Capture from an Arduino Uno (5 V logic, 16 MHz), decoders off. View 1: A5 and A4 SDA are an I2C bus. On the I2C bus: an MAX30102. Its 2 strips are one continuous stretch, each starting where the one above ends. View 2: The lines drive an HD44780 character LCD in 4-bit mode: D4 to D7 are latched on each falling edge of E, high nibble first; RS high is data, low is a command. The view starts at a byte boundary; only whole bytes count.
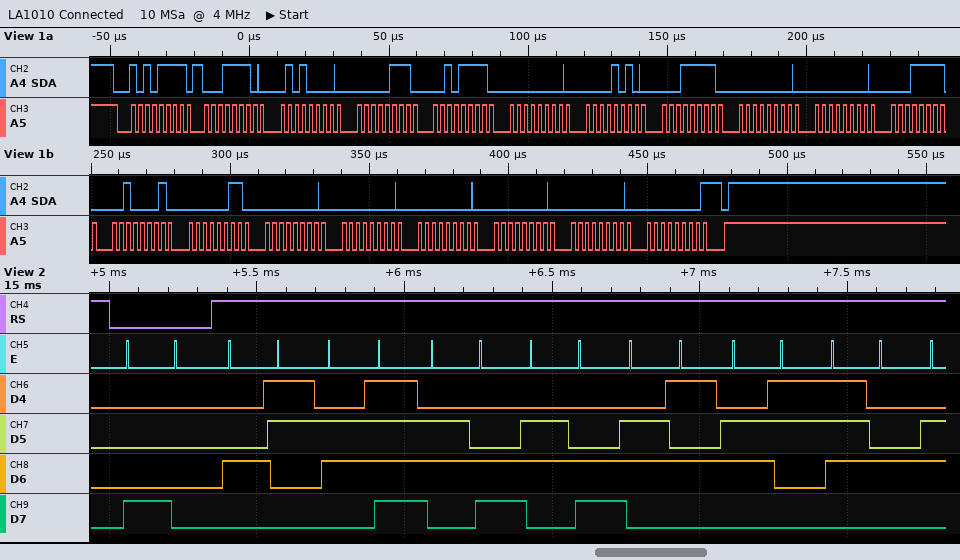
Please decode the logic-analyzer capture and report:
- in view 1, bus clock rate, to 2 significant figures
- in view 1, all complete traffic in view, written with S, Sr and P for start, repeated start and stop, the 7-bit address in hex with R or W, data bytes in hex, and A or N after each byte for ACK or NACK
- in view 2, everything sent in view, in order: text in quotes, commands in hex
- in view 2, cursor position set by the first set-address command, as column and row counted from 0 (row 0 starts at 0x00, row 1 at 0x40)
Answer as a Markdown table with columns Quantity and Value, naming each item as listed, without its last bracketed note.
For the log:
| Quantity | Value |
|---|---|
| in view 1, bus clock rate, to 2 significant figures | 400 kHz |
| in view 1, all complete traffic in view, written with S, Sr and P for start, repeated start and stop, the 7-bit address in hex with R or W, data bytes in hex, and A or N after each byte for ACK or NACK | S 57R A 1E A 50 A 07 A 2F A 00 A 0A A 1F A 00 A 00 A 1F A 21 A 03 A 00 A 00 A 00 A 00 A 00 A 00 N P |
| in view 2, everything sent in view, in order: text in quotes, commands in hex | 0x80 "Collect" |
| in view 2, cursor position set by the first set-address command, as column and row counted from 0 | column 0, row 0 |
